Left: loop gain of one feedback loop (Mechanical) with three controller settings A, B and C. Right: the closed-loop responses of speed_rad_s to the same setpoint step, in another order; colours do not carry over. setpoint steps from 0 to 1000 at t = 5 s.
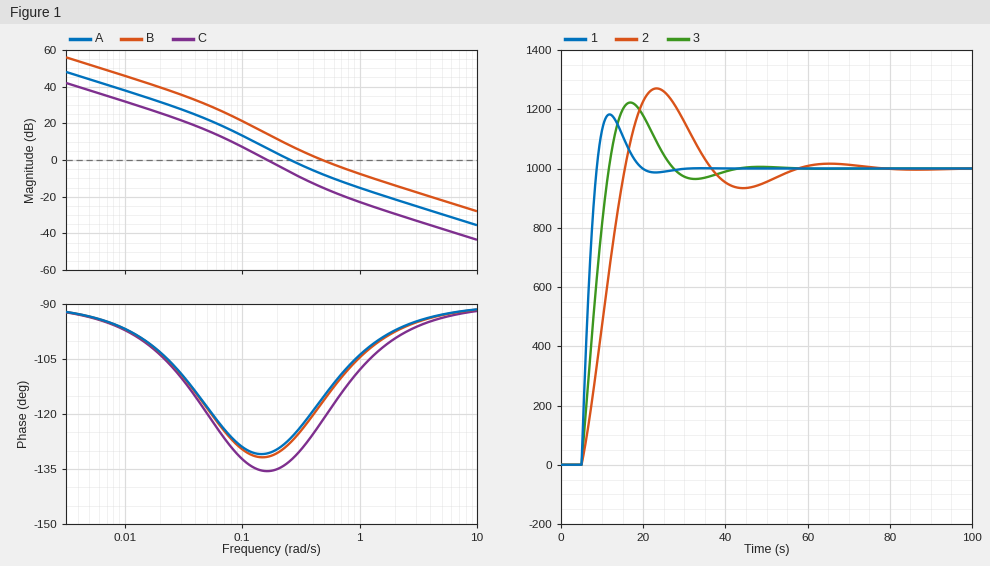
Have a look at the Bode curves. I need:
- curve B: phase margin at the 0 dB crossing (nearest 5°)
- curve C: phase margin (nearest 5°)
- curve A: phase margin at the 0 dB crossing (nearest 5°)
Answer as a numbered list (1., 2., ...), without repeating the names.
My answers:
1. 65°
2. 45°
3. 55°
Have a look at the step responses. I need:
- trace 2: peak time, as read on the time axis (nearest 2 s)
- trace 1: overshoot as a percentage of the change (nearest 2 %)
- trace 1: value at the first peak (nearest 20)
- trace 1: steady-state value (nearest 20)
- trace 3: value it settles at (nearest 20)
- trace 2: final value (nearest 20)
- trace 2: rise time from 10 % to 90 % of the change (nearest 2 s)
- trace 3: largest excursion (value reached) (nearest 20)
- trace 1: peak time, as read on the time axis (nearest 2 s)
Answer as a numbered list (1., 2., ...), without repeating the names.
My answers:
1. 24 s
2. 18 %
3. 1180
4. 1000
5. 1000
6. 1000
7. 8 s
8. 1220
9. 12 s
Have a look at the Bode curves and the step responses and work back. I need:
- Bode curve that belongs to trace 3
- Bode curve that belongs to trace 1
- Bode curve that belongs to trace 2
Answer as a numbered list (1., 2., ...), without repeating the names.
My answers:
1. A
2. B
3. C
